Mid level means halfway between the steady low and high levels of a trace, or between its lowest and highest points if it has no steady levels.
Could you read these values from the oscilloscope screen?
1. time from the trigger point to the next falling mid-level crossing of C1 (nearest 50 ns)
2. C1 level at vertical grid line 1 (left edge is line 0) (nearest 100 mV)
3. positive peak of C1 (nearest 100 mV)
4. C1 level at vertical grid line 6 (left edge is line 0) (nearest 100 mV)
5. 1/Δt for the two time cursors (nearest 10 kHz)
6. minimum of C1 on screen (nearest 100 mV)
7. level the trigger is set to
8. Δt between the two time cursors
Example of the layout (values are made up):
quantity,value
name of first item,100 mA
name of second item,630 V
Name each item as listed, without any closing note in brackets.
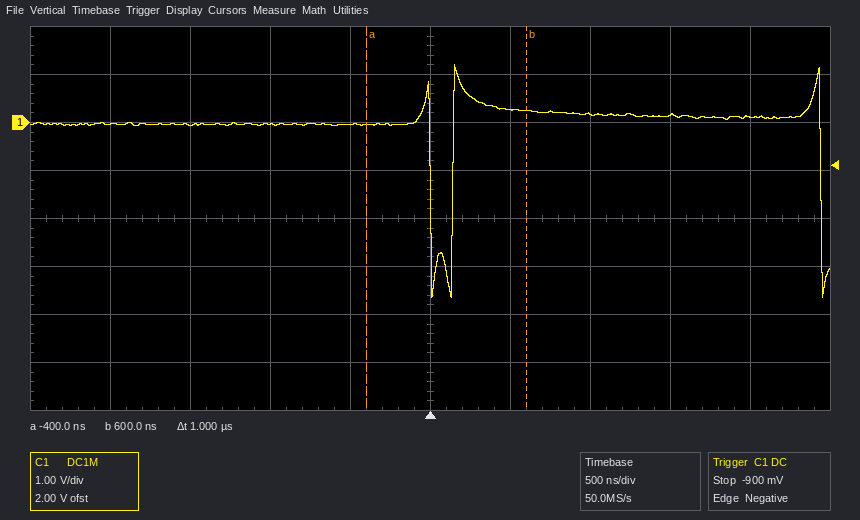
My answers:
quantity,value
time from the trigger point to the next falling mid-level crossing of C1,2.45 µs
C1 level at vertical grid line 1 (left edge is line 0),0.0 V
positive peak of C1,1.2 V
C1 level at vertical grid line 6 (left edge is line 0),300 mV
1/Δt for the two time cursors,1.00 MHz
minimum of C1 on screen,-3.6 V
level the trigger is set to,-900 mV
Δt between the two time cursors,1 µs
